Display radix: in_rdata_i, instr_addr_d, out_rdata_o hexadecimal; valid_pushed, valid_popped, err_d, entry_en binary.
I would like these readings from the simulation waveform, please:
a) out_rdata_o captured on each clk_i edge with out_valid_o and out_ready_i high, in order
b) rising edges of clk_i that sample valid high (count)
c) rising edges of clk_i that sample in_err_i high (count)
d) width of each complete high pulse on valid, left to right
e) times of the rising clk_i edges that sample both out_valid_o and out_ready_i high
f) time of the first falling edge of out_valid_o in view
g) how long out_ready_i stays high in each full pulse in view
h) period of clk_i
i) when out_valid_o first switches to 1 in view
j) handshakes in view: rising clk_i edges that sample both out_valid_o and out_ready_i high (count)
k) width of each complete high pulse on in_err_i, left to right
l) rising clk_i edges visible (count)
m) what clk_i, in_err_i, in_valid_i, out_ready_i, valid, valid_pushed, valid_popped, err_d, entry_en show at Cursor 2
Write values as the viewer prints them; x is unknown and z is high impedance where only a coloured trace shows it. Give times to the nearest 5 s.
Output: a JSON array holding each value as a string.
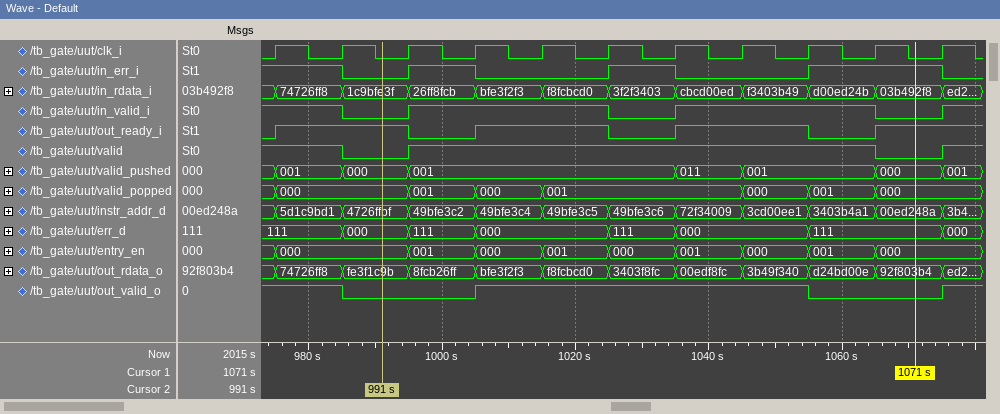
["74726ff8, bfe3f2f3, f8fcbcd0, 00edf8fc, 3b49f340", "9", "6", "70 s", "985 s, 1015 s, 1025 s, 1045 s, 1055 s", "985 s", "20 s, 20 s, 20 s", "10 s", "1005 s", "5", "10 s, 10 s, 20 s", "11", "clk_i=0, in_err_i=0, in_valid_i=0, out_ready_i=1, valid=0, valid_pushed=000, valid_popped=000, err_d=000, entry_en=000"]
